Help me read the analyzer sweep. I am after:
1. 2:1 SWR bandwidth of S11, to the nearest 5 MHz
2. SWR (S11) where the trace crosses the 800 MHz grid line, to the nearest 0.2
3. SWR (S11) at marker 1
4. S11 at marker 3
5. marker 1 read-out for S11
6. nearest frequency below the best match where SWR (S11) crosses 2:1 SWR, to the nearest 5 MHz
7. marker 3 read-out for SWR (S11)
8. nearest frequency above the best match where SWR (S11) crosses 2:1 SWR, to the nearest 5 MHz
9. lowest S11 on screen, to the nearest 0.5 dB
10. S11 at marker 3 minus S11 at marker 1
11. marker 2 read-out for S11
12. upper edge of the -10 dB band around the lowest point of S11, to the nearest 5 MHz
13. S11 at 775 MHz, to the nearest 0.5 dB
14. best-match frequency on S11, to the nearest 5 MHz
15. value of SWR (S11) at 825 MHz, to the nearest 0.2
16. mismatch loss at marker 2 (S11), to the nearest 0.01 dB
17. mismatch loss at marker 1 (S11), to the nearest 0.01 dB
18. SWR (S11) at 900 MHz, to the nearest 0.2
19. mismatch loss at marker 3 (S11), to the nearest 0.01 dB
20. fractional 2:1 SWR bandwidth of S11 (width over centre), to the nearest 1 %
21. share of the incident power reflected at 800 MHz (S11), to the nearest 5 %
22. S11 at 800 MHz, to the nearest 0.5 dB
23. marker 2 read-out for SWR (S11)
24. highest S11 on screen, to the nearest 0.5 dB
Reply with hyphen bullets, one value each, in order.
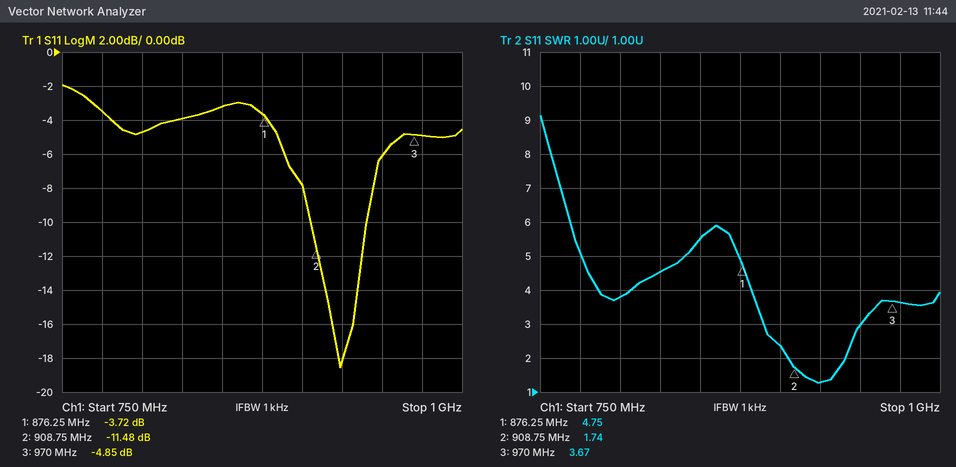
- 35 MHz
- 3.8
- 4.75
- -4.85 dB
- -3.72 dB
- 905 MHz
- 3.67
- 940 MHz
- -18.5 dB
- -1.13 dB
- -11.48 dB
- 940 MHz
- -3.5 dB
- 925 MHz
- 4.6
- 0.32 dB
- 2.40 dB
- 2.4
- 1.72 dB
- 4 %
- 35 %
- -4.5 dB
- 1.74
- -2.0 dB
